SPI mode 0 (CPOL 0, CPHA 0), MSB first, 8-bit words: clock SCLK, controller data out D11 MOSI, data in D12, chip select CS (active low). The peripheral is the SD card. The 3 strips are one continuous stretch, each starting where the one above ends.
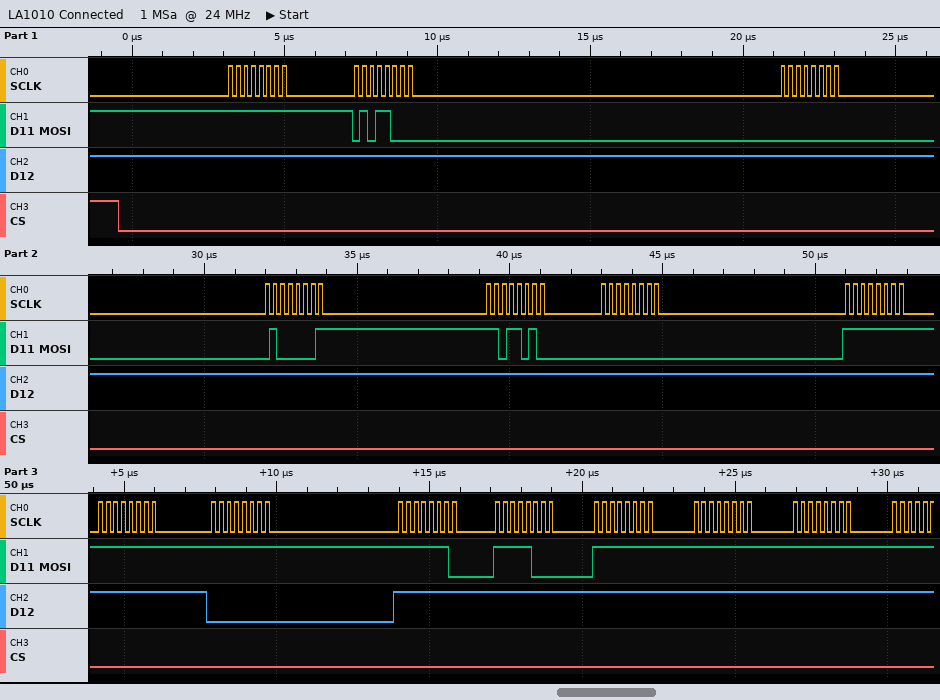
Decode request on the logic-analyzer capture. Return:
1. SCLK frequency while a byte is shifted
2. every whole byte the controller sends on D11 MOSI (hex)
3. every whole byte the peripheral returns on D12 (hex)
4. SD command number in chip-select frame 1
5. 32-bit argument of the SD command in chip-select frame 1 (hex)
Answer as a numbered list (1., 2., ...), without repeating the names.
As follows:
1. 4 MHz
2. 0xFF 0x58 0x00 0x41 0xDA 0x00 0xFF 0xFF 0xFF 0xFE 0xF8 0xFF 0xFF 0xFF
3. 0xFF 0xFF 0xFF 0xFF 0xFF 0xFF 0xFF 0xFF 0x00 0xFF 0xFF 0xFF 0xFF 0xFF
4. CMD24
5. 0x0041DA00
